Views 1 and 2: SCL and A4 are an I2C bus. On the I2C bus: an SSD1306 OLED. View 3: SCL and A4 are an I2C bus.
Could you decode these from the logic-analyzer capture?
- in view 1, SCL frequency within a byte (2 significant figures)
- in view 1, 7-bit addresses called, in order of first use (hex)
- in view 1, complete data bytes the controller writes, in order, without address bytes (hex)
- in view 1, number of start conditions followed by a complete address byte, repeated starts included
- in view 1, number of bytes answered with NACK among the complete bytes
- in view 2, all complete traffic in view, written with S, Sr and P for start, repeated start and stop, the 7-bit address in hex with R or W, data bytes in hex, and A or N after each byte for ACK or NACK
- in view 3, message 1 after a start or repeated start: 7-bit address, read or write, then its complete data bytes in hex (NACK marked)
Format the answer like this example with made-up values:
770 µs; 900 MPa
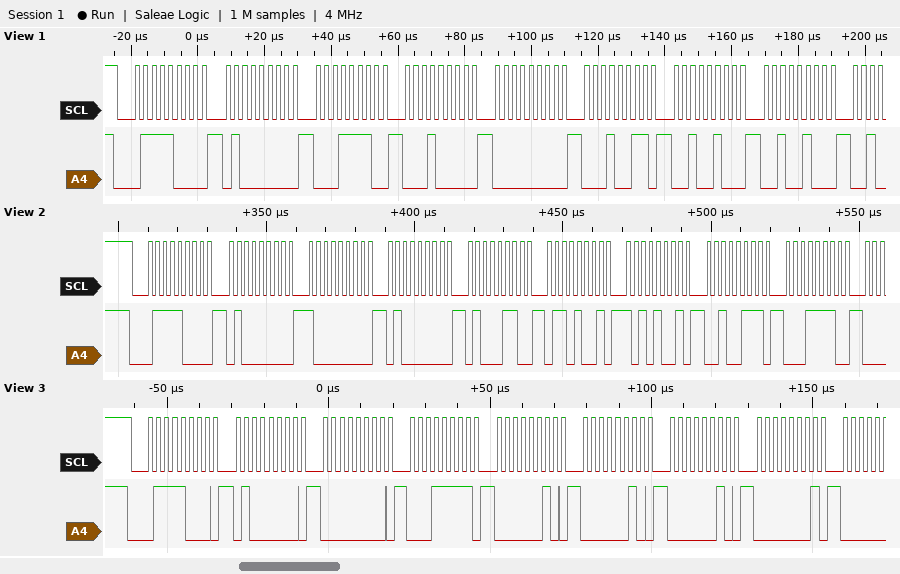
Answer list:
400 kHz; 0x3C; 40 1E 10 00 13 24 24; 1; 0; S 3CW A 40 A 80 A 40 A 46 A 69 A A9 A 27 A 1E A; 0x3C write: 40 00 1F 02 02 02 01
